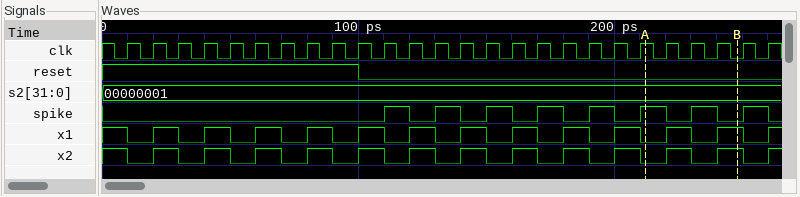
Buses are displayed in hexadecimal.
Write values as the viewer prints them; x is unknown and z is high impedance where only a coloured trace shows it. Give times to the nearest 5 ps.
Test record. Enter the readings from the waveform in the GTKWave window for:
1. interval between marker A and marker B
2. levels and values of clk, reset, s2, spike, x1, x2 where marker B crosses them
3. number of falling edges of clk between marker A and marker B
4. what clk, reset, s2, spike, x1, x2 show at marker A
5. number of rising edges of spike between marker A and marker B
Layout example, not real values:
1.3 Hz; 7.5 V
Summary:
35 ps; clk=0, reset=0, s2=00000001, spike=0, x1=1, x2=1; 4; clk=1, reset=0, s2=00000001, spike=1, x1=0, x2=0; 1
